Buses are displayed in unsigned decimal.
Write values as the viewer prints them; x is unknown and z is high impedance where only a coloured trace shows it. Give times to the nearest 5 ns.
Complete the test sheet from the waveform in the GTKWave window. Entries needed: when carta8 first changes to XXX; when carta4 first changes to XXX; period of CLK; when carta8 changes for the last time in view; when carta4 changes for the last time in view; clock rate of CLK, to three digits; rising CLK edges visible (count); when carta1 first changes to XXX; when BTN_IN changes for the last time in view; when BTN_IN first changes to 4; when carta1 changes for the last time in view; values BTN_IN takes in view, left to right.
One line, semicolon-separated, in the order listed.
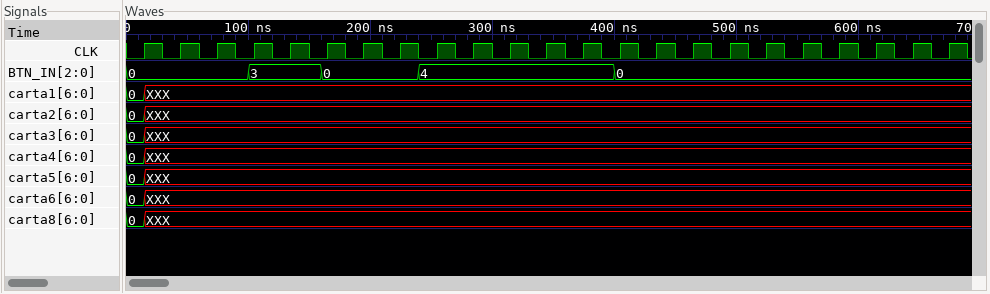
15 ns; 15 ns; 30 ns; 15 ns; 15 ns; 33.3 MHz; 23; 15 ns; 400 ns; 240 ns; 15 ns; 0, 3, 0, 4, 0
